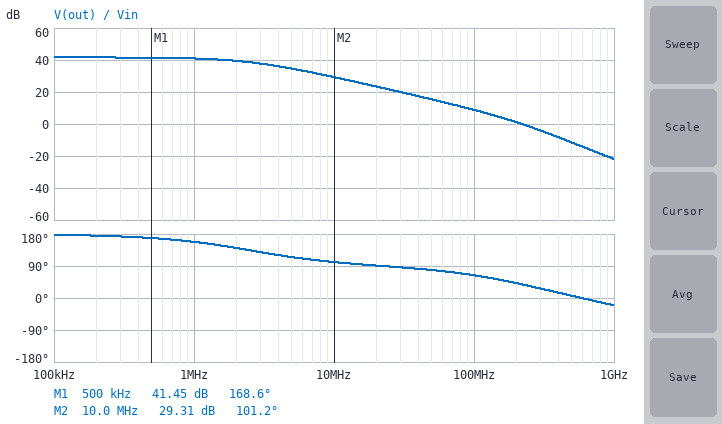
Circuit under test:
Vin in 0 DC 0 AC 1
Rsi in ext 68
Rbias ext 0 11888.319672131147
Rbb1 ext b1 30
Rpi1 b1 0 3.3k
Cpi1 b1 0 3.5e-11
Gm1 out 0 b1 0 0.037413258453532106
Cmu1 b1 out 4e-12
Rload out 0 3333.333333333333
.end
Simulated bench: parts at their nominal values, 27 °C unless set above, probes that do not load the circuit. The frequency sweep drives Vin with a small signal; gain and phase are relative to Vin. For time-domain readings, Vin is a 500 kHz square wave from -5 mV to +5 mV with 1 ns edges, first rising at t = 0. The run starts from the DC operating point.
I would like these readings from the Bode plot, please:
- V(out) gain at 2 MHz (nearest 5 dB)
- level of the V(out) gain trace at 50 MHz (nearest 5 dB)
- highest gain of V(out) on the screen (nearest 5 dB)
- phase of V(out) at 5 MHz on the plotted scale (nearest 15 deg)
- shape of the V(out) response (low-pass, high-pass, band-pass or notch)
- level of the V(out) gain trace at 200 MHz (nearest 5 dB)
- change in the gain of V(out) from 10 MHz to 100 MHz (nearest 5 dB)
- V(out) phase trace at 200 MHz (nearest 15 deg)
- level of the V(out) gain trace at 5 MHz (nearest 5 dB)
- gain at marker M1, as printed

40 dB
15 dB
40 dB
120 deg
low-pass
0 dB
-20 dB
45 deg
35 dB
41.45 dB
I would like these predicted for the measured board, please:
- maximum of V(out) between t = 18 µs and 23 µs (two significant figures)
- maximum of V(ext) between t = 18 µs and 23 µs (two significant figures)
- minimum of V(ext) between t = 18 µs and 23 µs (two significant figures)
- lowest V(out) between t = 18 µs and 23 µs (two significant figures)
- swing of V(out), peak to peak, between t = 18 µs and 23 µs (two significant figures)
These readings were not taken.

600 mV
4.9 mV
-4.9 mV
-600 mV
1.2 V
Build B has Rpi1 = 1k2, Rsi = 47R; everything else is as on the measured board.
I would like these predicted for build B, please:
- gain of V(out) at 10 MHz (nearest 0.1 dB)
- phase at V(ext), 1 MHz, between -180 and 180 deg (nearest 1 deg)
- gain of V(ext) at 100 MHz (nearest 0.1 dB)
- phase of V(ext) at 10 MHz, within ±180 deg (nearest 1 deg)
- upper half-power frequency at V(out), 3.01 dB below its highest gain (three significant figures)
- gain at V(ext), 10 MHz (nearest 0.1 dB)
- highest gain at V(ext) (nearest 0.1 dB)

30.7 dB
-8 deg
-5.8 dB
-13 deg
3.09 MHz
-4.7 dB
-0.4 dB
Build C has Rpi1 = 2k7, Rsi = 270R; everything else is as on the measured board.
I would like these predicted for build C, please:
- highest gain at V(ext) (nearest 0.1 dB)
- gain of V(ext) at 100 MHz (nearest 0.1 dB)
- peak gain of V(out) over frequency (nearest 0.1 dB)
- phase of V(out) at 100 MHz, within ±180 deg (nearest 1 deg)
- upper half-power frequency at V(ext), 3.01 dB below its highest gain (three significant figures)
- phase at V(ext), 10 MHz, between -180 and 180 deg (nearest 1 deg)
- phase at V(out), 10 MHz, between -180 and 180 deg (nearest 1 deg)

-1.0 dB
-16.2 dB
40.8 dB
60 deg
1.06 MHz
-24 deg
93 deg
